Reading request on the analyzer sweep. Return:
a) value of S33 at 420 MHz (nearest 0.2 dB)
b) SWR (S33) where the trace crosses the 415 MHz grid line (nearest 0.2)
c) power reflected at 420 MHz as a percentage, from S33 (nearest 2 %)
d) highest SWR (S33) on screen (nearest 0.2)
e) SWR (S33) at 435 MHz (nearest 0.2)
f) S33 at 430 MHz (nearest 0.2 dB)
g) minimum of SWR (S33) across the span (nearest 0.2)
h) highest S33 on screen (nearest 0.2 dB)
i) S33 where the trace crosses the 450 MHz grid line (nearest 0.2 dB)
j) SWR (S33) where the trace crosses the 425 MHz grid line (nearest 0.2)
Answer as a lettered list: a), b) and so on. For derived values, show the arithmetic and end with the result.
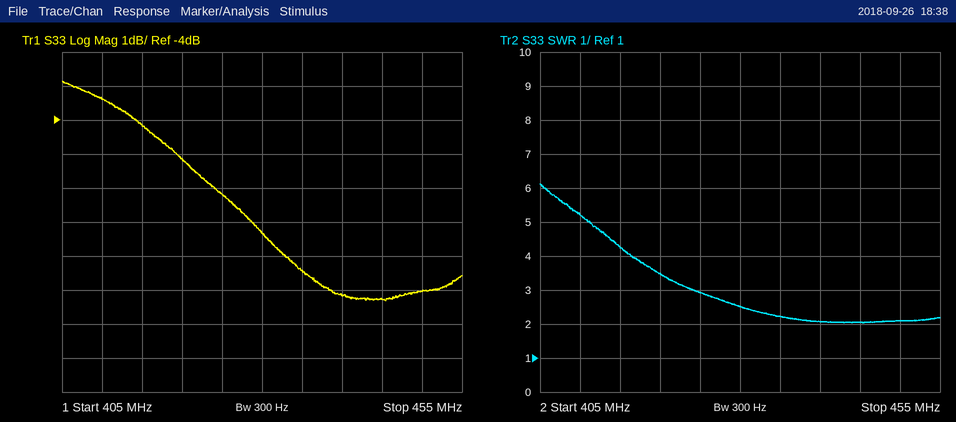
a) -5.2 dB
b) 4.2
c) 10^(-5.2/10) ≈ 30 %
d) 6.2
e) 2.2
f) -7.4 dB
g) 2.0
h) -2.8 dB
i) -9.0 dB
j) 3.0
